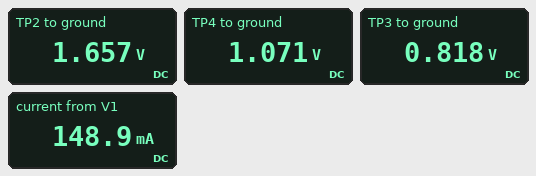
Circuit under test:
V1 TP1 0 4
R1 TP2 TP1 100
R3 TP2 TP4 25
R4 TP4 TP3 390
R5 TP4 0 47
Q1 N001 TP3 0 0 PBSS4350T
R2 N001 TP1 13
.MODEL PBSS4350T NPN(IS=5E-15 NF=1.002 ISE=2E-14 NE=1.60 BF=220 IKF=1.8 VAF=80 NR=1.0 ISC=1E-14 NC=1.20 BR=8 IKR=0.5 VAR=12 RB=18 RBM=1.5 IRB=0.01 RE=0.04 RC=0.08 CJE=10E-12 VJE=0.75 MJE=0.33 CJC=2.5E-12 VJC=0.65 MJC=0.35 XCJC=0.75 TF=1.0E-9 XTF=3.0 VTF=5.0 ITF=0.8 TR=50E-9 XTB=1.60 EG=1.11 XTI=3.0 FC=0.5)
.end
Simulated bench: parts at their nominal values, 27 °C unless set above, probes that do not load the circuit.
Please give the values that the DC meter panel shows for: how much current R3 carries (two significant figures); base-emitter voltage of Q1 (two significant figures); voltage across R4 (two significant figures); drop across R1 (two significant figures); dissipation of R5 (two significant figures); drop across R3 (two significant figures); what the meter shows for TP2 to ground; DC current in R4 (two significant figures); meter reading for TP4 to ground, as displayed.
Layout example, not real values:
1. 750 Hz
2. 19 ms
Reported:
1. 23 mA
2. 820 mV
3. 250 mV
4. 2.3 V
5. 24 mW
6. 590 mV
7. 1.657 V
8. 650 µA
9. 1.071 V
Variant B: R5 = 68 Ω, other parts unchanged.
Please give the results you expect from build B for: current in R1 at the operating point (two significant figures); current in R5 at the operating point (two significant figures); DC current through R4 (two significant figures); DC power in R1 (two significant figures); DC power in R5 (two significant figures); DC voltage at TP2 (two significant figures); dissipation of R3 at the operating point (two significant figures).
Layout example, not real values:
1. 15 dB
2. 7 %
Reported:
1. 21 mA
2. 20 mA
3. 1.3 mA
4. 45 mW
5. 27 mW
6. 1.9 V
7. 11 mW
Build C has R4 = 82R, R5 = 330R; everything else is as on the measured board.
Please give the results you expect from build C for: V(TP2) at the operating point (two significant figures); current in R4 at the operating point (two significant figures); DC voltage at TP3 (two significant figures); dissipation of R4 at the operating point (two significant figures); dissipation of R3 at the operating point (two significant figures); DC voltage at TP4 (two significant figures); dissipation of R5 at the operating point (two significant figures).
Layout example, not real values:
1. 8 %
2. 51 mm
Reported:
1. 2.3 V
2. 11 mA
3. 960 mV
4. 10 mW
5. 7.2 mW
6. 1.9 V
7. 11 mW
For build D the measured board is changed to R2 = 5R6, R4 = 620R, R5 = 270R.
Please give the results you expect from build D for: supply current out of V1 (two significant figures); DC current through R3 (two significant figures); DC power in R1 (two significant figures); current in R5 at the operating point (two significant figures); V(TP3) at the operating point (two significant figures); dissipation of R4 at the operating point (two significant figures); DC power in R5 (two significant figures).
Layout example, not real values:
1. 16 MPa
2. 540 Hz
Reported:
1. 440 mA
2. 12 mA
3. 14 mW
4. 9.3 mA
5. 890 mV
6. 4.2 mW
7. 23 mW
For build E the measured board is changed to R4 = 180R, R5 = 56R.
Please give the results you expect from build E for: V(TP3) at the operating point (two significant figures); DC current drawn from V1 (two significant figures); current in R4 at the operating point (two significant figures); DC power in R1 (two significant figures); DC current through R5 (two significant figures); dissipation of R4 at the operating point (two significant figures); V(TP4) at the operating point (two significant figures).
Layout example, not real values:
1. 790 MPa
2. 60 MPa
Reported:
1. 860 mV
2. 310 mA
3. 1.7 mA
4. 51 mW
5. 21 mA
6. 530 µW
7. 1.2 V
